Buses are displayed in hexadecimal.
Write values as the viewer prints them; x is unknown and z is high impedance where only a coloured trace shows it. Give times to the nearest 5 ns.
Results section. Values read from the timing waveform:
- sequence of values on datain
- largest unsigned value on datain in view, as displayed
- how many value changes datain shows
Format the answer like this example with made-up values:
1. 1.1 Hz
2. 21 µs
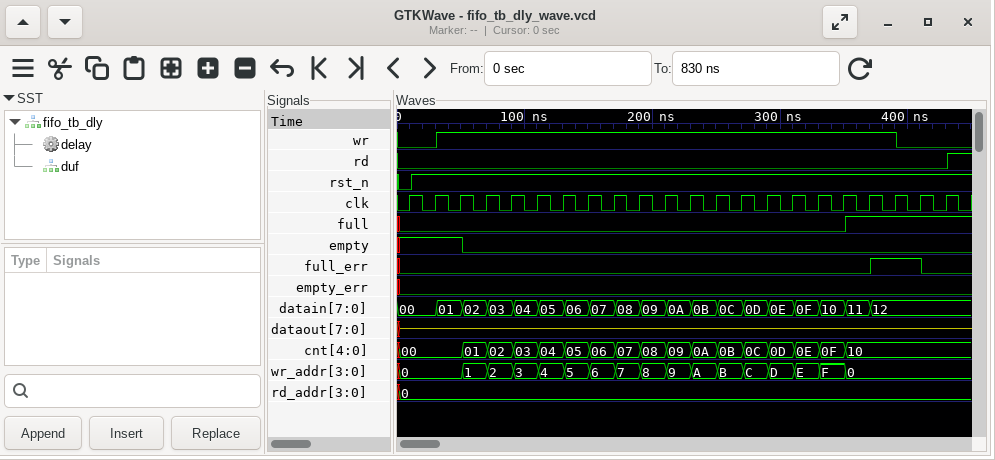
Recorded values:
1. 00, 01, 02, 03, 04, 05, 06, 07, 08, 09, 0A, 0B, 0C, 0D, 0E, 0F, 10, 11, 12
2. 12
3. 18
